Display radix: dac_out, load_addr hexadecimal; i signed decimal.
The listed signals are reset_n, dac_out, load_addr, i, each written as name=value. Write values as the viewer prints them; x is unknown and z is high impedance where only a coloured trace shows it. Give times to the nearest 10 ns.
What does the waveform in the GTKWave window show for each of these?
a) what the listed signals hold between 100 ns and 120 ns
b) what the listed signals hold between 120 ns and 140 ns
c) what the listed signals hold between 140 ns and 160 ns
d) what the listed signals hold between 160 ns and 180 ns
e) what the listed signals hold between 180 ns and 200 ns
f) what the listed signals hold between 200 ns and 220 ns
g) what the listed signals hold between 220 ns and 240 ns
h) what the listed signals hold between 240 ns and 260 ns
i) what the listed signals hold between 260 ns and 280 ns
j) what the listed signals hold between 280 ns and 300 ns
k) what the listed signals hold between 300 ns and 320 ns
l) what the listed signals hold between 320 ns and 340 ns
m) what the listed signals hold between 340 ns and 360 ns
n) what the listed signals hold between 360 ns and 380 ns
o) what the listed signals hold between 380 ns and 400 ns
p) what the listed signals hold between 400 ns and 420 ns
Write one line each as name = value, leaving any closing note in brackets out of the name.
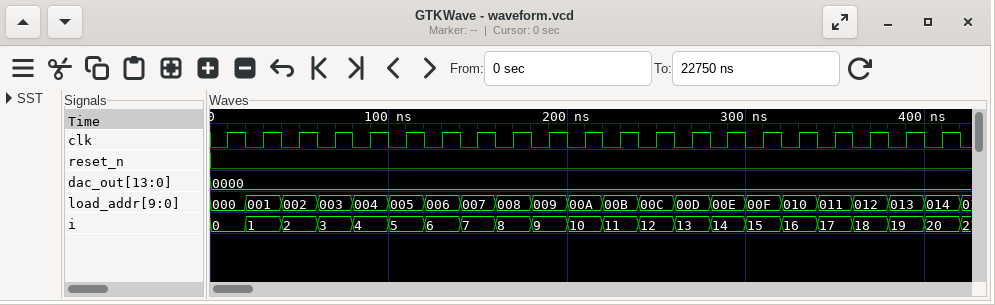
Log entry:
what the listed signals hold between 100 ns and 120 ns = reset_n=0, dac_out=0000, load_addr=005, i=5
what the listed signals hold between 120 ns and 140 ns = reset_n=0, dac_out=0000, load_addr=006, i=6
what the listed signals hold between 140 ns and 160 ns = reset_n=0, dac_out=0000, load_addr=007, i=7
what the listed signals hold between 160 ns and 180 ns = reset_n=0, dac_out=0000, load_addr=008, i=8
what the listed signals hold between 180 ns and 200 ns = reset_n=0, dac_out=0000, load_addr=009, i=9
what the listed signals hold between 200 ns and 220 ns = reset_n=0, dac_out=0000, load_addr=00A, i=10
what the listed signals hold between 220 ns and 240 ns = reset_n=0, dac_out=0000, load_addr=00B, i=11
what the listed signals hold between 240 ns and 260 ns = reset_n=0, dac_out=0000, load_addr=00C, i=12
what the listed signals hold between 260 ns and 280 ns = reset_n=0, dac_out=0000, load_addr=00D, i=13
what the listed signals hold between 280 ns and 300 ns = reset_n=0, dac_out=0000, load_addr=00E, i=14
what the listed signals hold between 300 ns and 320 ns = reset_n=0, dac_out=0000, load_addr=00F, i=15
what the listed signals hold between 320 ns and 340 ns = reset_n=0, dac_out=0000, load_addr=010, i=16
what the listed signals hold between 340 ns and 360 ns = reset_n=0, dac_out=0000, load_addr=011, i=17
what the listed signals hold between 360 ns and 380 ns = reset_n=0, dac_out=0000, load_addr=012, i=18
what the listed signals hold between 380 ns and 400 ns = reset_n=0, dac_out=0000, load_addr=013, i=19
what the listed signals hold between 400 ns and 420 ns = reset_n=0, dac_out=0000, load_addr=014, i=20
